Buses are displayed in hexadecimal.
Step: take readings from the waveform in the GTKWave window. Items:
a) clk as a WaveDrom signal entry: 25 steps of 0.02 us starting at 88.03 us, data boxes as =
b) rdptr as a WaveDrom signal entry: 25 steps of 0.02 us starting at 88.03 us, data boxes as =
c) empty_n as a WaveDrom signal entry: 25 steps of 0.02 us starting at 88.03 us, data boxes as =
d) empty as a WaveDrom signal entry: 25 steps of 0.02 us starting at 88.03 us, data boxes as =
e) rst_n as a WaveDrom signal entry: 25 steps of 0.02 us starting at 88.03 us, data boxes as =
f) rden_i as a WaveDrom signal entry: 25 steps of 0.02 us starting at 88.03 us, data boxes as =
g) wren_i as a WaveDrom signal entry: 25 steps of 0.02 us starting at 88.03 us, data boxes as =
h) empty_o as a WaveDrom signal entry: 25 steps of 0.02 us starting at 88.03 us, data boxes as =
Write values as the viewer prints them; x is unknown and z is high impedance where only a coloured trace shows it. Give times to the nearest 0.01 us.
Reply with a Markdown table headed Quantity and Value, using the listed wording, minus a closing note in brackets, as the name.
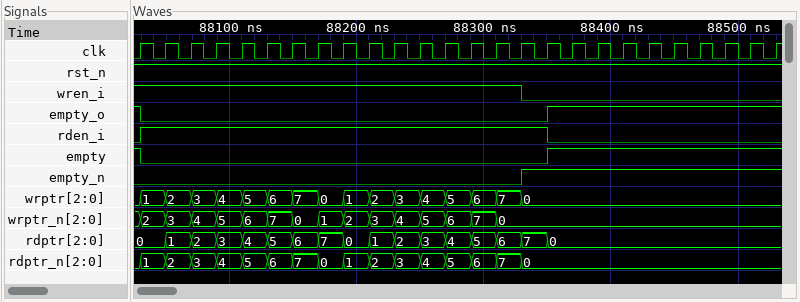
| Quantity | Value |
|---|---|
| clk as a WaveDrom signal entry: 25 steps of 0.02 us starting at 88.03 us, data boxes as = | {name: 'clk', wave: 'p........................'} |
| rdptr as a WaveDrom signal entry: 25 steps of 0.02 us starting at 88.03 us, data boxes as = | {name: 'rdptr', wave: '=================........', data: '0 1 2 3 4 5 6 7 0 1 2 3 4 5 6 7 0'} |
| empty_n as a WaveDrom signal entry: 25 steps of 0.02 us starting at 88.03 us, data boxes as = | {name: 'empty_n', wave: '0..............1.........'} |
| empty as a WaveDrom signal entry: 25 steps of 0.02 us starting at 88.03 us, data boxes as = | {name: 'empty', wave: '0...............1........'} |
| rst_n as a WaveDrom signal entry: 25 steps of 0.02 us starting at 88.03 us, data boxes as = | {name: 'rst_n', wave: '1........................'} |
| rden_i as a WaveDrom signal entry: 25 steps of 0.02 us starting at 88.03 us, data boxes as = | {name: 'rden_i', wave: '1...............0........'} |
| wren_i as a WaveDrom signal entry: 25 steps of 0.02 us starting at 88.03 us, data boxes as = | {name: 'wren_i', wave: '1..............0.........'} |
| empty_o as a WaveDrom signal entry: 25 steps of 0.02 us starting at 88.03 us, data boxes as = | {name: 'empty_o', wave: '0...............1........'} |
